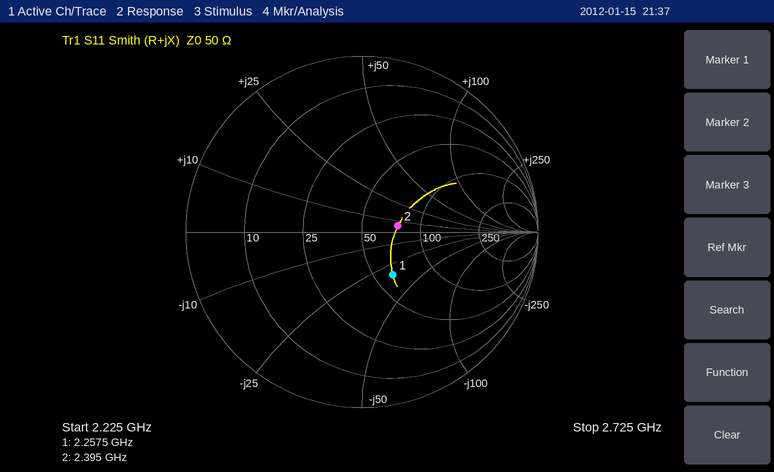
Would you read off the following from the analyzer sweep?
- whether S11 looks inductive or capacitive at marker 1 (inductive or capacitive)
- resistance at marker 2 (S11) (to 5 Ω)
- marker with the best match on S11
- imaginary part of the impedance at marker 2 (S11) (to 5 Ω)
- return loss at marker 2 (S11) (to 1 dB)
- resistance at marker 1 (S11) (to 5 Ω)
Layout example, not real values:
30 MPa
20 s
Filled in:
capacitive
75 Ω
marker 2
+5 Ω
14 dB
60 Ω
